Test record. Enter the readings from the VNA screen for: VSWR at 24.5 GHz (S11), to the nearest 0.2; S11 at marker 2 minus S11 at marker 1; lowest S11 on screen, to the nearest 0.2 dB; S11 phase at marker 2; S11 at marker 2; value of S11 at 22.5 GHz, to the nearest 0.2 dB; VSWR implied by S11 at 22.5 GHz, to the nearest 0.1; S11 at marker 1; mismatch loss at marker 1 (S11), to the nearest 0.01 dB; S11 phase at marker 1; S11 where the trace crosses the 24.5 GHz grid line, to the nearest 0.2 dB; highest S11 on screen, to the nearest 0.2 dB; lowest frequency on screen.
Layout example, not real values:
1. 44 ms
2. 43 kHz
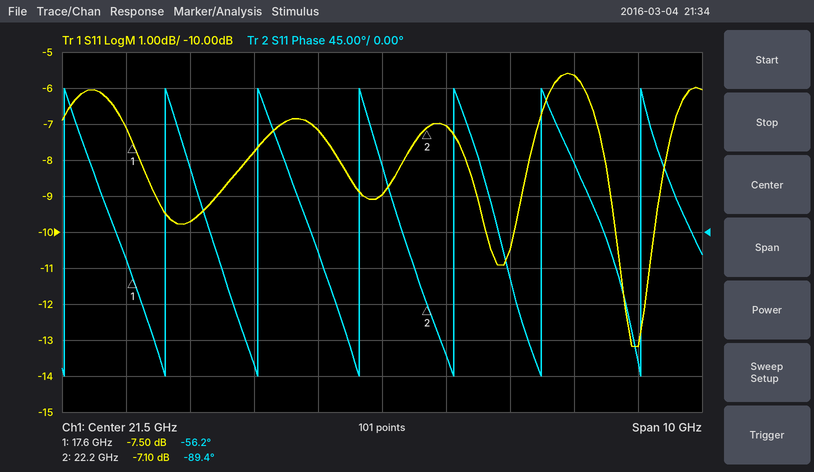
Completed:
1. 3.2
2. 0.40 dB
3. -13.2 dB
4. -89.4°
5. -7.10 dB
6. -7.0 dB
7. 2.6
8. -7.50 dB
9. 0.85 dB
10. -56.2°
11. -5.6 dB
12. -5.6 dB
13. 16.5 GHz
